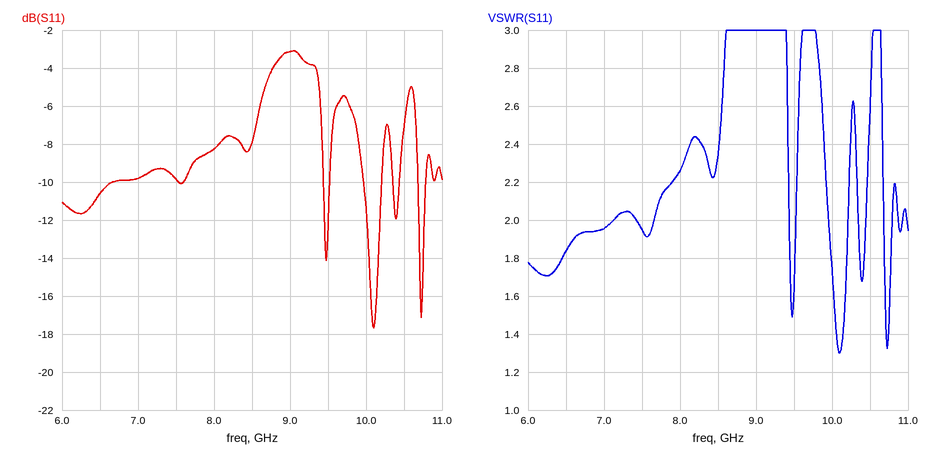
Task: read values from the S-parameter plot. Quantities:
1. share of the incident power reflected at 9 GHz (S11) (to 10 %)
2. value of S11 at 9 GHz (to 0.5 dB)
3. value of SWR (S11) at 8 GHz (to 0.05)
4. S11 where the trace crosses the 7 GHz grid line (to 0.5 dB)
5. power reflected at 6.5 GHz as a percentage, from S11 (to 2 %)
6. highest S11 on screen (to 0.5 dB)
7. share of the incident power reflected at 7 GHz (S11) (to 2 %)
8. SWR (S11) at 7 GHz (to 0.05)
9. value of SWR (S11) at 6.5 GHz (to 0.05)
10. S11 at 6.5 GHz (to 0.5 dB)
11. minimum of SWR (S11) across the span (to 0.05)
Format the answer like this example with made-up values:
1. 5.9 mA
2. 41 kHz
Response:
1. 50 %
2. -3.0 dB
3. 2.25
4. -10.0 dB
5. 8 %
6. -3.0 dB
7. 10 %
8. 1.95
9. 1.85
10. -10.5 dB
11. 1.30
